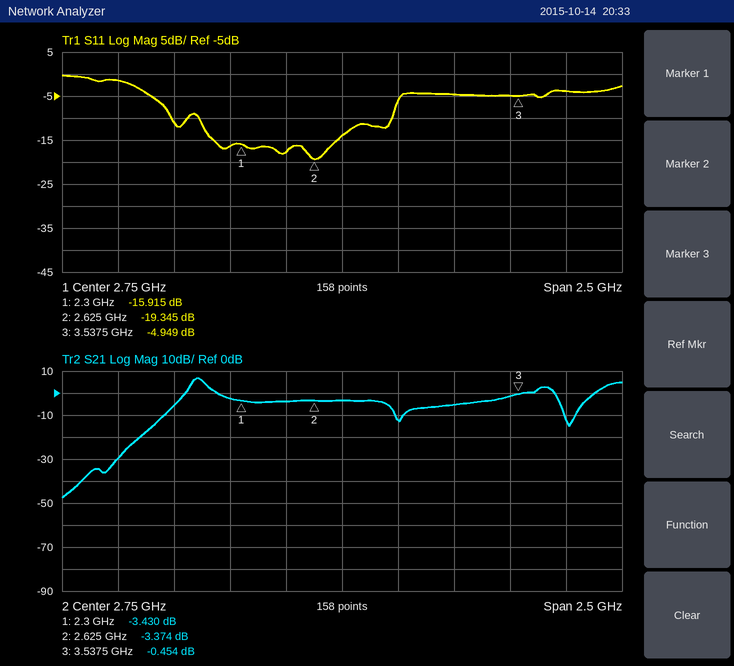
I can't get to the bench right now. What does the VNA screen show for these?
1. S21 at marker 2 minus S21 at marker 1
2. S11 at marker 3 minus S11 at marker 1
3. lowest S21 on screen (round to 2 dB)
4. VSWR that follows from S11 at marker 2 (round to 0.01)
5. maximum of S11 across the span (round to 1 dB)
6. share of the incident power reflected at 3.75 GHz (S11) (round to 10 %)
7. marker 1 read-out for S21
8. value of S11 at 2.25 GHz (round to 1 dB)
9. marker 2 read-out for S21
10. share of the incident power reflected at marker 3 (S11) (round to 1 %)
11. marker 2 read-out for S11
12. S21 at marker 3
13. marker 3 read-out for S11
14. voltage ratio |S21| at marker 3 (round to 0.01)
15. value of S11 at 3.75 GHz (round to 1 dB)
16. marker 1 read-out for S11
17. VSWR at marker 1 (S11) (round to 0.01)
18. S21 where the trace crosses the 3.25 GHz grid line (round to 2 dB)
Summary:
0.056 dB
10.966 dB
-48 dB
1.24
0 dB
40 %
-3.430 dB
-16 dB
-3.374 dB
32 %
-19.345 dB
-0.454 dB
-4.949 dB
0.95
-4 dB
-15.915 dB
1.38
-6 dB
